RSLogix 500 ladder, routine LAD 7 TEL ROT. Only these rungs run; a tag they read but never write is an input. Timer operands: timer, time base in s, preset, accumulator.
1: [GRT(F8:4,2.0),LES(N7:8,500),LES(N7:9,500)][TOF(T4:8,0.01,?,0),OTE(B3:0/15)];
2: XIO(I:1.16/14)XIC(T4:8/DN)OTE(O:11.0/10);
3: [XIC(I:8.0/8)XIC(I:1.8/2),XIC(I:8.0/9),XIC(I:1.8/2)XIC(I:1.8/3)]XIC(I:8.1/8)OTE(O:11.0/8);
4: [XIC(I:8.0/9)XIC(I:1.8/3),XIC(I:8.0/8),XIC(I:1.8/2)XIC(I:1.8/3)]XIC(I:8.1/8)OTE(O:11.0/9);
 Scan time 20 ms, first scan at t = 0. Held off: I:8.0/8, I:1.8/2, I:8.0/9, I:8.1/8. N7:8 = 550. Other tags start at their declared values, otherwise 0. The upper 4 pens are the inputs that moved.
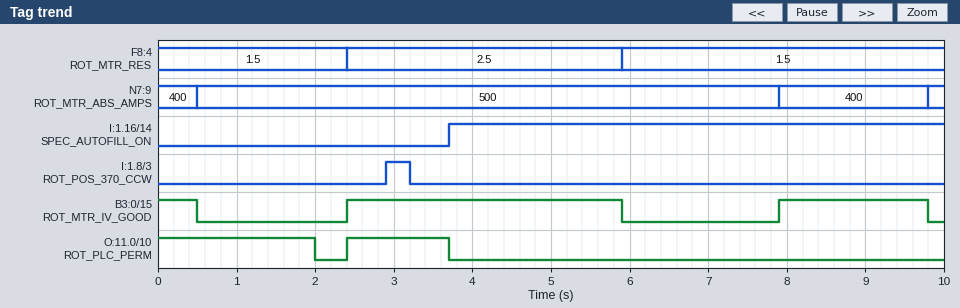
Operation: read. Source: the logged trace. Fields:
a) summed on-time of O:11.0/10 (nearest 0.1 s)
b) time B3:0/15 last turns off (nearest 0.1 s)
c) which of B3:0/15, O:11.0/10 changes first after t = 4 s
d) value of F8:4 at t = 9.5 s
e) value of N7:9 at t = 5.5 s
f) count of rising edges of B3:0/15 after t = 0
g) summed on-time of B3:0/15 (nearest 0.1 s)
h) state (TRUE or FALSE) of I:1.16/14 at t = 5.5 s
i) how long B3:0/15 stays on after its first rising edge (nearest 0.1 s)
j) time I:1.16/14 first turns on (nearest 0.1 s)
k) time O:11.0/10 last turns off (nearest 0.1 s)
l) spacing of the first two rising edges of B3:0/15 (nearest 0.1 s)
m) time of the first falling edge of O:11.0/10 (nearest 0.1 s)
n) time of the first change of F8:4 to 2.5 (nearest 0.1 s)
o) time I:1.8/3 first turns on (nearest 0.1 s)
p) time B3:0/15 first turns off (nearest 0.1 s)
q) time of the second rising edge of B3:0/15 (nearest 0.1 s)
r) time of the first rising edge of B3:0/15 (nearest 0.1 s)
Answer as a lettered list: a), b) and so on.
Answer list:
a) 3.3 s
b) 9.8 s
c) B3:0/15
d) 1.5
e) 500
f) 2
g) 5.9 s
h) TRUE
i) 3.5 s
j) 3.7 s
k) 3.7 s
l) 5.5 s
m) 2.0 s
n) 2.4 s
o) 2.9 s
p) 0.5 s
q) 7.9 s
r) 2.4 s
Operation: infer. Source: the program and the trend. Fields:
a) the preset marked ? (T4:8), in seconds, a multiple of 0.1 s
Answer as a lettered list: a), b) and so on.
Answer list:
a) 1.5 s
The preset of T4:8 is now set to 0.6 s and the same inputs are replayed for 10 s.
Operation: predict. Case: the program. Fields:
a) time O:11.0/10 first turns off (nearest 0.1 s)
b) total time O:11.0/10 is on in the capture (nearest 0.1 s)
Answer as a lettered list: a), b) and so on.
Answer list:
a) 1.1 s
b) 2.4 s
